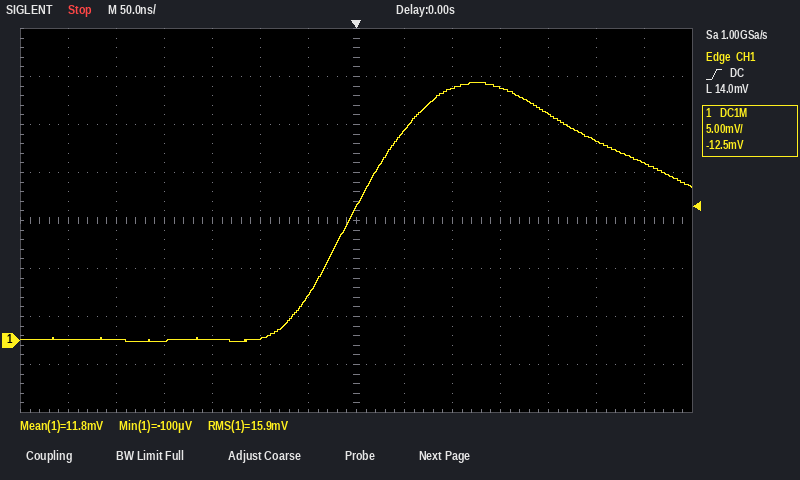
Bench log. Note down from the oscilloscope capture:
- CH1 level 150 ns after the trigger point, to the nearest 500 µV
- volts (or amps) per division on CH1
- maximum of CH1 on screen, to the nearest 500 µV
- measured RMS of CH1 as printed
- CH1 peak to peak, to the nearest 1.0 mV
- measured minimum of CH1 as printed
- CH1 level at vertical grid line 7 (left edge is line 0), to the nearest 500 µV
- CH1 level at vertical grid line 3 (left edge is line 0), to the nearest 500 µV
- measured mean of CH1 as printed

26.5 mV
5 mV
27.0 mV
15.9 mV
27.0 mV
-100 µV
14.0 mV
0.0 mV
11.8 mV
